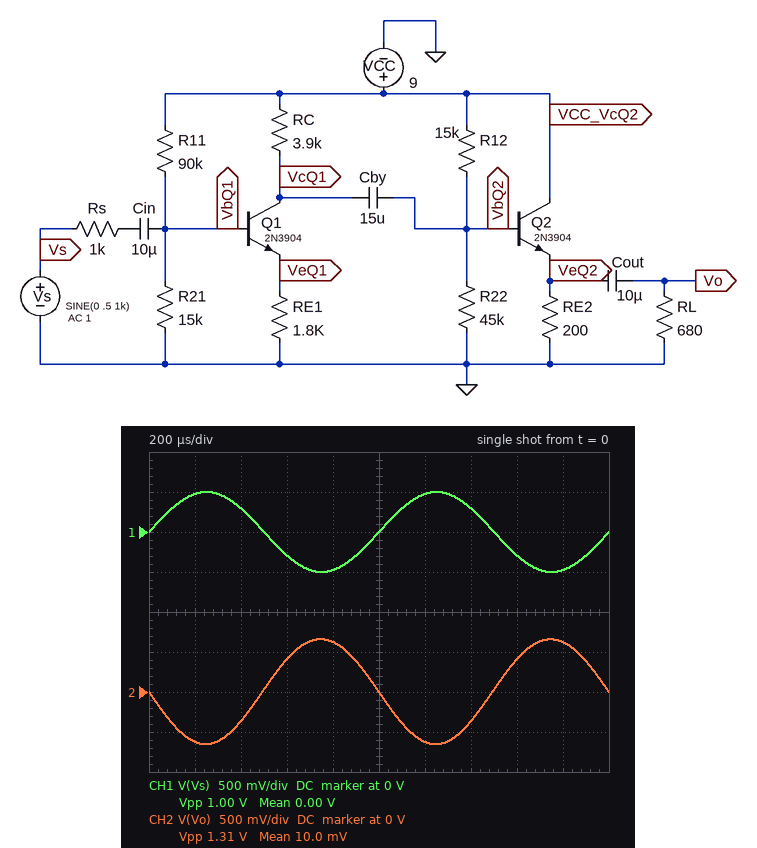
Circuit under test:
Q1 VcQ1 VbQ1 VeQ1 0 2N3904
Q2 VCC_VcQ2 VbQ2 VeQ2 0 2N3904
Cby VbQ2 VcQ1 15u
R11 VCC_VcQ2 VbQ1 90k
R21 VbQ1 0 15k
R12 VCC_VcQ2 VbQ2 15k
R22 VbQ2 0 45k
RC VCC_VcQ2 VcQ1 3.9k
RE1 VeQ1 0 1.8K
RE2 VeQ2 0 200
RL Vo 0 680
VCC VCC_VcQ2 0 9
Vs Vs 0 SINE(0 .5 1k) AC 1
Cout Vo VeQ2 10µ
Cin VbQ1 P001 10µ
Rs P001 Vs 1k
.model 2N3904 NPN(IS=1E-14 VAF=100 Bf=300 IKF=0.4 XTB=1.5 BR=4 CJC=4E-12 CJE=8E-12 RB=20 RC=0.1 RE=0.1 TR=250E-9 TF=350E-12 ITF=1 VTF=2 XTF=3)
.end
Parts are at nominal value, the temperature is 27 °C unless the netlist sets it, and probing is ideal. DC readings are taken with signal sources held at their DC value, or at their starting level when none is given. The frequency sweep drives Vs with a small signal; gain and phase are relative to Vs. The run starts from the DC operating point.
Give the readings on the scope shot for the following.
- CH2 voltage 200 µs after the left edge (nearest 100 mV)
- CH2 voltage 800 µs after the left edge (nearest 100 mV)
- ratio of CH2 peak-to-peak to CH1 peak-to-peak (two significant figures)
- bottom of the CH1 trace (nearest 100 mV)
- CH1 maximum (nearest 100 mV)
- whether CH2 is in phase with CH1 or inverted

-600 mV
600 mV
1.3
-500 mV
500 mV
inverted
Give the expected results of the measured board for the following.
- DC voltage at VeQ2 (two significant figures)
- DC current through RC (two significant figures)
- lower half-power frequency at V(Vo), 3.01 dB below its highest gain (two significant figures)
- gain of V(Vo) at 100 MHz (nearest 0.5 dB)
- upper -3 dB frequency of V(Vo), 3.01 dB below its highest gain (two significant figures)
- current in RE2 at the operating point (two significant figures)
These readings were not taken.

5.0 V
360 µA
23 Hz
-14.0 dB
7.7 MHz
25 mA
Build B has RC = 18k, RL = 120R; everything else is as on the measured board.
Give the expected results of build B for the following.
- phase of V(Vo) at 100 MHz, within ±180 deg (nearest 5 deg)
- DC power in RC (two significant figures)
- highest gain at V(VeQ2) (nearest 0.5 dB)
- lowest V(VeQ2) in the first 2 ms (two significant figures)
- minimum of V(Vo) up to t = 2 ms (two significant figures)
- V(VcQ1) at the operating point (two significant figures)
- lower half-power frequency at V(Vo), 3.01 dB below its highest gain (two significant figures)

-30 deg
2.3 mW
9.5 dB
3.7 V
-1.2 V
2.6 V
110 Hz
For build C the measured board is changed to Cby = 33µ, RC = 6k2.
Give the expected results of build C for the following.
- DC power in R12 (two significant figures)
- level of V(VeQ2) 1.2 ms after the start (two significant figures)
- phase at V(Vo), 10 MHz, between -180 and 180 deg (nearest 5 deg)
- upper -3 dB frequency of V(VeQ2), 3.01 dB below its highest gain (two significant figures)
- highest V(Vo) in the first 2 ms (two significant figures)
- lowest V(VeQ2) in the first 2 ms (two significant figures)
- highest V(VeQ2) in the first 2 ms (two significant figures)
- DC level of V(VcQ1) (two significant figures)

690 µW
4.2 V
95 deg
5.5 MHz
890 mV
4.1 V
5.9 V
6.8 V
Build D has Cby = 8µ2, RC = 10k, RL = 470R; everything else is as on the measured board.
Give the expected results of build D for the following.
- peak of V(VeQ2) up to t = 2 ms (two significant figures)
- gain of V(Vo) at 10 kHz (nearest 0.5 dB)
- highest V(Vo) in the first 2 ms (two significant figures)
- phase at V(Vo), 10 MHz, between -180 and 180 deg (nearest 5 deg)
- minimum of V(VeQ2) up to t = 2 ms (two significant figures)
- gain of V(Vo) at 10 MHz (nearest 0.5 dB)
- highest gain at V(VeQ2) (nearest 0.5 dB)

6.1 V
7.0 dB
1.1 V
90 deg
3.9 V
-1.0 dB
7.5 dB
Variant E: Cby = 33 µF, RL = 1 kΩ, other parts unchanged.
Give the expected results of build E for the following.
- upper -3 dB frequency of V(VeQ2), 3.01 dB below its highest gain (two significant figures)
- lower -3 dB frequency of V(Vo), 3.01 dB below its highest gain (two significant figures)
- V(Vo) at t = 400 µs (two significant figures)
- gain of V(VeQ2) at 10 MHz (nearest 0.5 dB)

7.8 MHz
16 Hz
-370 mV
-1.5 dB
